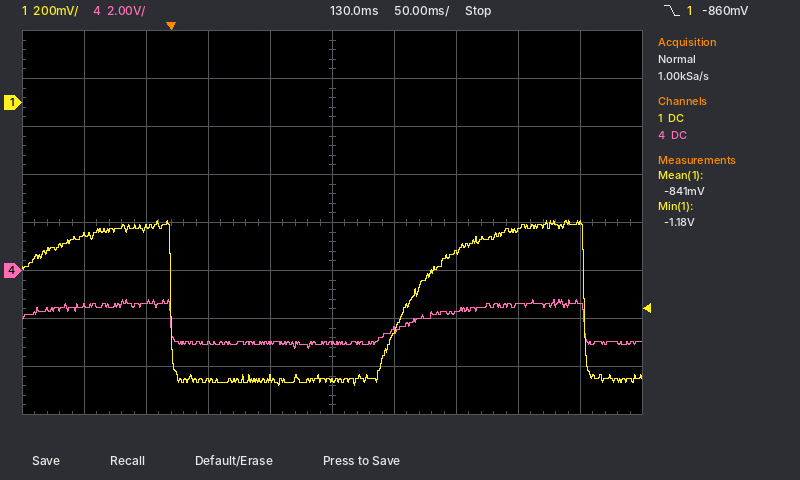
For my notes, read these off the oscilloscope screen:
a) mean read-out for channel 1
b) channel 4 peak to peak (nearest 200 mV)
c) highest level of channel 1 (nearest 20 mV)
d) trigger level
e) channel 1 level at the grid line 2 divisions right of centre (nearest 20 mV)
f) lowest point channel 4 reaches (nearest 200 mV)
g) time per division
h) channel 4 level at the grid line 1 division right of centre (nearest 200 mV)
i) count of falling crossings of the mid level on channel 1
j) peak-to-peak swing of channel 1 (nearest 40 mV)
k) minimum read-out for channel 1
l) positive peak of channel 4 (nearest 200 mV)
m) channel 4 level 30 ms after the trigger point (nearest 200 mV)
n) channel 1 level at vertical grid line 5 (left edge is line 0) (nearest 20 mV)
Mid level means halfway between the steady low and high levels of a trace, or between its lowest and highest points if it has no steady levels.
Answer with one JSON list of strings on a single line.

["-841 mV", "2.0 V", "-500 mV", "-860 mV", "-620 mV", "-3.2 V", "50 ms", "-2.4 V", "2", "680 mV", "-1.18 V", "-1.2 V", "-3.0 V", "-1.16 V"]
